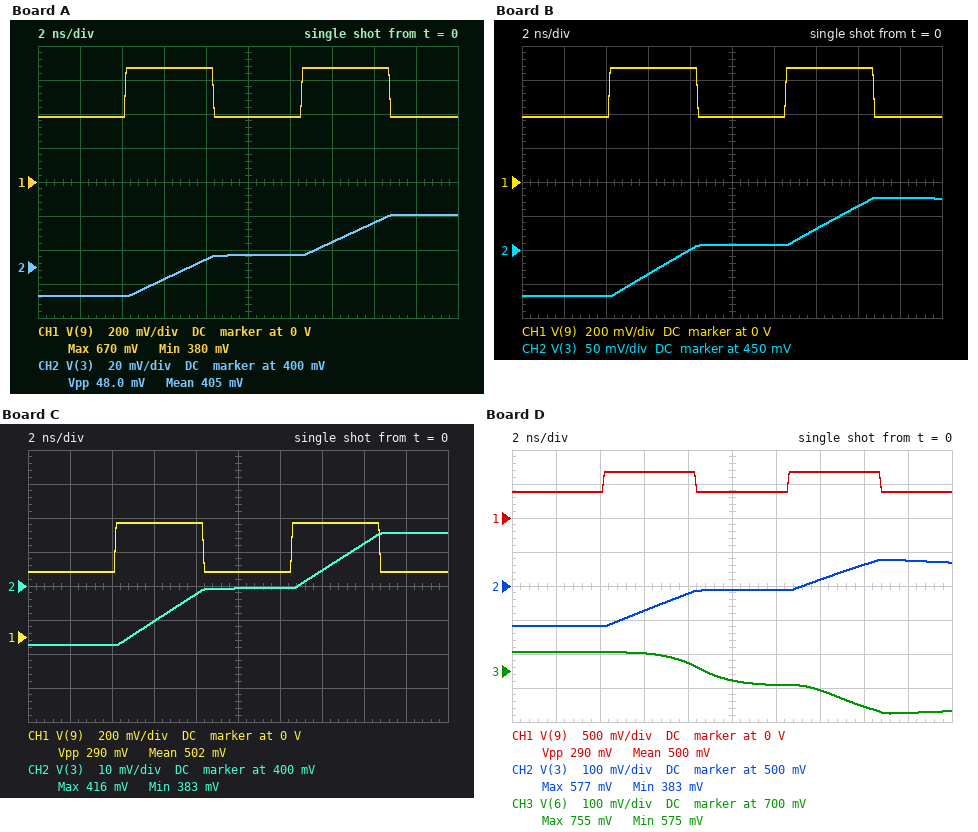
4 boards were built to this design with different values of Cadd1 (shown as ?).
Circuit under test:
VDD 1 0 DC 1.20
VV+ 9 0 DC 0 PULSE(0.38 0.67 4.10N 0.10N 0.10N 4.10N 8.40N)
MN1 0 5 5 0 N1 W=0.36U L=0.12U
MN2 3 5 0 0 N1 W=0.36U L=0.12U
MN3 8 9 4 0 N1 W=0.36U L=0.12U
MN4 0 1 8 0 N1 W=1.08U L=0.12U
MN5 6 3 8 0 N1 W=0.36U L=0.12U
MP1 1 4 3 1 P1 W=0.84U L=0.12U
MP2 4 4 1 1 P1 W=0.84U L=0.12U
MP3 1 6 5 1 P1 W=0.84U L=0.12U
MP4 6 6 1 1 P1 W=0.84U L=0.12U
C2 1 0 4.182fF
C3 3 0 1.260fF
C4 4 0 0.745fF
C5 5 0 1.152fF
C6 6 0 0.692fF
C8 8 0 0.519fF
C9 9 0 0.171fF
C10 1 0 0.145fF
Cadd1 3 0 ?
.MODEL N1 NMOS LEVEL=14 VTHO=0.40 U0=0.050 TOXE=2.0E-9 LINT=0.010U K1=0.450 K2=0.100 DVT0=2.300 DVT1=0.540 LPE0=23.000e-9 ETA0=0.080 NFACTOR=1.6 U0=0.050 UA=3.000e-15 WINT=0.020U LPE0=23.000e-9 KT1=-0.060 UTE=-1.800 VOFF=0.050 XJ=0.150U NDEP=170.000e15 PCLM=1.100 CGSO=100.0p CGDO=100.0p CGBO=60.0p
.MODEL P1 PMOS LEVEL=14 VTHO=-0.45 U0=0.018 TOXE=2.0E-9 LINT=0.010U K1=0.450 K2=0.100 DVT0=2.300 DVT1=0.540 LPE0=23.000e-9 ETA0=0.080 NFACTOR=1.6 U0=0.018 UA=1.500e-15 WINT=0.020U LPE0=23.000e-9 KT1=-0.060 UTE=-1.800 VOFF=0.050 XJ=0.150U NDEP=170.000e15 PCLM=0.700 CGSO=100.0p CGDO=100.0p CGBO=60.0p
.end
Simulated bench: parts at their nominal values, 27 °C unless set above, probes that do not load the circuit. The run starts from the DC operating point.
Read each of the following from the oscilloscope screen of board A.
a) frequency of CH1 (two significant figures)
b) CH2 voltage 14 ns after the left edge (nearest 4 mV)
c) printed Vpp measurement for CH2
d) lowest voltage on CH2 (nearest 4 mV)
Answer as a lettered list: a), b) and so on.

a) 120 MHz
b) 416 mV
c) 48.0 mV
d) 384 mV
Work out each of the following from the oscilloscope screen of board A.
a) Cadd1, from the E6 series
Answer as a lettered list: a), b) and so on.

a) 1.5 pF
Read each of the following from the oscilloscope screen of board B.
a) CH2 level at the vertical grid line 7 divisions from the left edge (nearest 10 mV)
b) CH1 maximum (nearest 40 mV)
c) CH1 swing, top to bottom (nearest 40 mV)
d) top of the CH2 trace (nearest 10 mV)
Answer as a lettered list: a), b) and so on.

a) 480 mV
b) 680 mV
c) 280 mV
d) 530 mV
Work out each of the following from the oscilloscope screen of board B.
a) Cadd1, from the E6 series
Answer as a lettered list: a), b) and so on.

a) 470 fF
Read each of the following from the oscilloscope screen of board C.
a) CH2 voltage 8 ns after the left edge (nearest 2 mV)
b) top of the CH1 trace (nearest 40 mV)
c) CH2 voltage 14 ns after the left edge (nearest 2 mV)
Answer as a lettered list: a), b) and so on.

a) 398 mV
b) 680 mV
c) 404 mV
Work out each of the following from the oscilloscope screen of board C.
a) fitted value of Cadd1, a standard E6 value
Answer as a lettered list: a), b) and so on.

a) 2.2 pF
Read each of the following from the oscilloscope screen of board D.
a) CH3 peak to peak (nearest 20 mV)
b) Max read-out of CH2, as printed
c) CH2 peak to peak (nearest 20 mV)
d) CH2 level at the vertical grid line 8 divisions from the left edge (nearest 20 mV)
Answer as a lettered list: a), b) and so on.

a) 180 mV
b) 577 mV
c) 200 mV
d) 560 mV
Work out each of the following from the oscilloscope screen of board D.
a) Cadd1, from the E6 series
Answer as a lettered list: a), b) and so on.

a) 330 fF
